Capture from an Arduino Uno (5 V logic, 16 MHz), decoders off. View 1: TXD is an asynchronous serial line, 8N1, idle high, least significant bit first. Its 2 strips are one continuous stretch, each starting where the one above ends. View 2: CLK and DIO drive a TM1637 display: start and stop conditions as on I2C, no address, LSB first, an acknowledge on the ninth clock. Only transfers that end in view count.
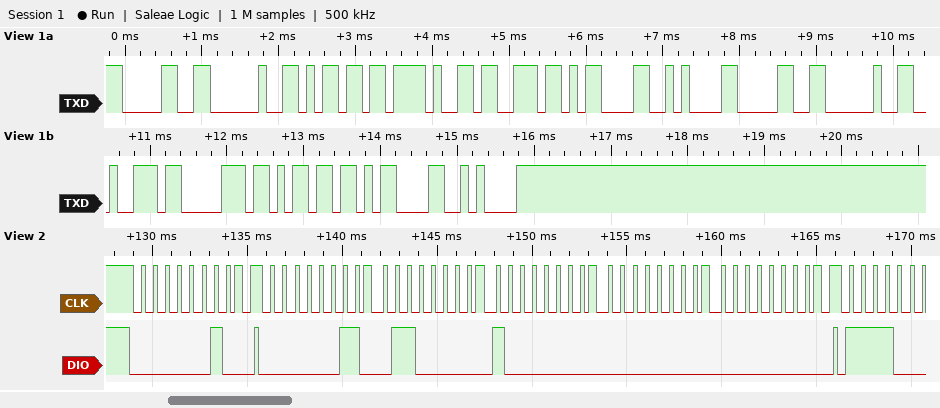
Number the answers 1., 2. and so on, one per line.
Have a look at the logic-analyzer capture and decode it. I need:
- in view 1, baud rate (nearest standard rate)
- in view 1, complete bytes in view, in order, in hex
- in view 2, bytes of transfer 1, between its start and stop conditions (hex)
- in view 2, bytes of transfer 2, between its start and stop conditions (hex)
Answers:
1. 9600 baud
2. 30 20 6D 2F 73 0D 0A 30 20 72 70 6D 0D 0A
3. 40
4. C0 06 01 00 00
